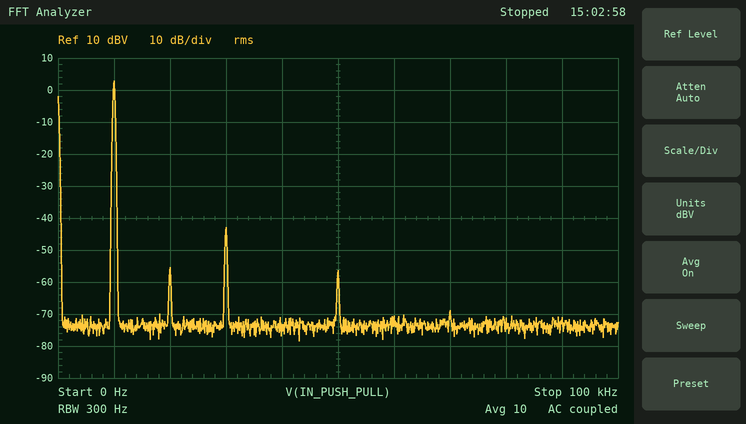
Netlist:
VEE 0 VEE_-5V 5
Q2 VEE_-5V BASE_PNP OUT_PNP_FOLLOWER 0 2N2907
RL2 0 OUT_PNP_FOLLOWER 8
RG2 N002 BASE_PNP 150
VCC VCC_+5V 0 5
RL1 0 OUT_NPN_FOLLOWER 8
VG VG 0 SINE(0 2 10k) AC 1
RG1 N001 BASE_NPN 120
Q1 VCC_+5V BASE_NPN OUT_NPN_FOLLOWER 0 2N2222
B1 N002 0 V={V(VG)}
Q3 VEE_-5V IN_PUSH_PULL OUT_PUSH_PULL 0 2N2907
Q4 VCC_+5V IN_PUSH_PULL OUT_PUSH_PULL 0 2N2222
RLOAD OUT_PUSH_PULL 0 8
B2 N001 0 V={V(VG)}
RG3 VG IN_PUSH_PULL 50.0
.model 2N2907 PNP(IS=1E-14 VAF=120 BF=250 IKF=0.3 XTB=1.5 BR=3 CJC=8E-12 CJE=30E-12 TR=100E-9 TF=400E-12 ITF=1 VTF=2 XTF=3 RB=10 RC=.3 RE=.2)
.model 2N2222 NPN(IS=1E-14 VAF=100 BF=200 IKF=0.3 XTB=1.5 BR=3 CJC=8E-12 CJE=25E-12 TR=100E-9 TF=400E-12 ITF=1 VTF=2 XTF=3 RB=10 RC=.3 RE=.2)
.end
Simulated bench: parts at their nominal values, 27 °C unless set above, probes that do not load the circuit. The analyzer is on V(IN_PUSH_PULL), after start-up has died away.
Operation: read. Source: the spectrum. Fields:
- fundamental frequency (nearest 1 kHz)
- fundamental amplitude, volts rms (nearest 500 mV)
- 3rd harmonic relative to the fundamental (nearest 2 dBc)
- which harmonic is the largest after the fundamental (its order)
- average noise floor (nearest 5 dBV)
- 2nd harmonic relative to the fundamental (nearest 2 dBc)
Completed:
10 kHz
1.5 V
-46 dBc
3
-75 dBV
-58 dBc
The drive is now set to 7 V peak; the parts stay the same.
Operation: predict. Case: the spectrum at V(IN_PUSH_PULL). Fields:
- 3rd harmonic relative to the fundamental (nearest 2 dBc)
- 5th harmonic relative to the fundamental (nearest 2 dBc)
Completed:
-26 dBc
-34 dBc
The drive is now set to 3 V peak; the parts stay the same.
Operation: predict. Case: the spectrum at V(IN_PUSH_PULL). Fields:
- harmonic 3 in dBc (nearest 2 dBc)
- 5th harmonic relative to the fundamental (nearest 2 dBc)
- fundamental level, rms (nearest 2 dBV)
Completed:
-44 dBc
-56 dBc
6 dBV
